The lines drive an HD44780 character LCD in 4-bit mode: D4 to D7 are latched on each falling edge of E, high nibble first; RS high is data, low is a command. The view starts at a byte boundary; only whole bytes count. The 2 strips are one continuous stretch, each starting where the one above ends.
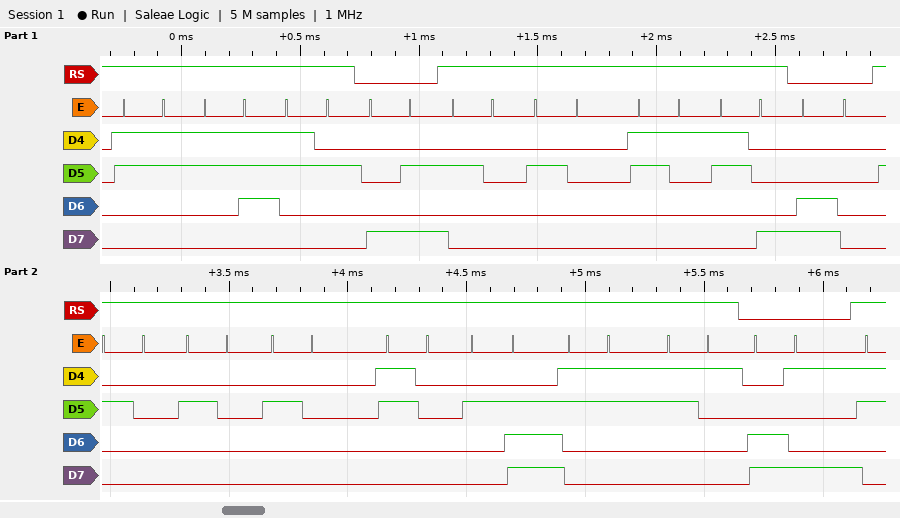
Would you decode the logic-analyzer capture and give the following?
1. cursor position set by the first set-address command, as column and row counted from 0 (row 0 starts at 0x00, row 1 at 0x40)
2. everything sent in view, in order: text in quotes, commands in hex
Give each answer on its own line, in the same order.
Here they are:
column 10, row 0
"372" 0x8A "  18" 0xC0 "   0.31" 0xC9
